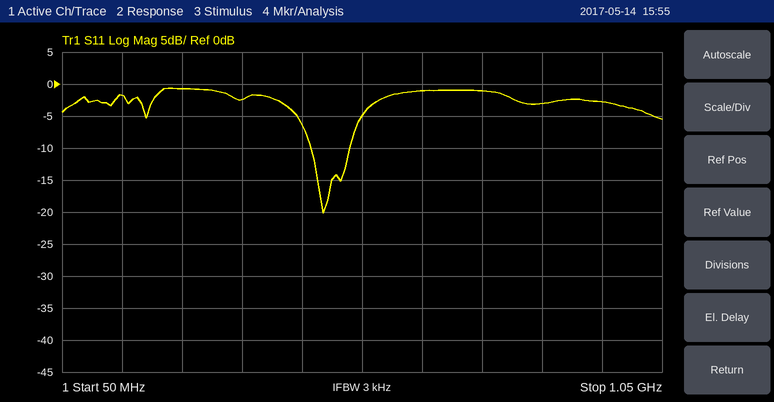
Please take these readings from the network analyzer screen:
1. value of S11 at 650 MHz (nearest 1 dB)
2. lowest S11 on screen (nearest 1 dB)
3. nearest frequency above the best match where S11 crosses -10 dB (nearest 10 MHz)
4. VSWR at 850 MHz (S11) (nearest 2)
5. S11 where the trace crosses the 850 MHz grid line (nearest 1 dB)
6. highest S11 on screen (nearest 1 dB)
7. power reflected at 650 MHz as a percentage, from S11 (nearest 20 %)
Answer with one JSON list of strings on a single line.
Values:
["-1 dB", "-20 dB", "530 MHz", "6", "-3 dB", "-1 dB", "80 %"]
